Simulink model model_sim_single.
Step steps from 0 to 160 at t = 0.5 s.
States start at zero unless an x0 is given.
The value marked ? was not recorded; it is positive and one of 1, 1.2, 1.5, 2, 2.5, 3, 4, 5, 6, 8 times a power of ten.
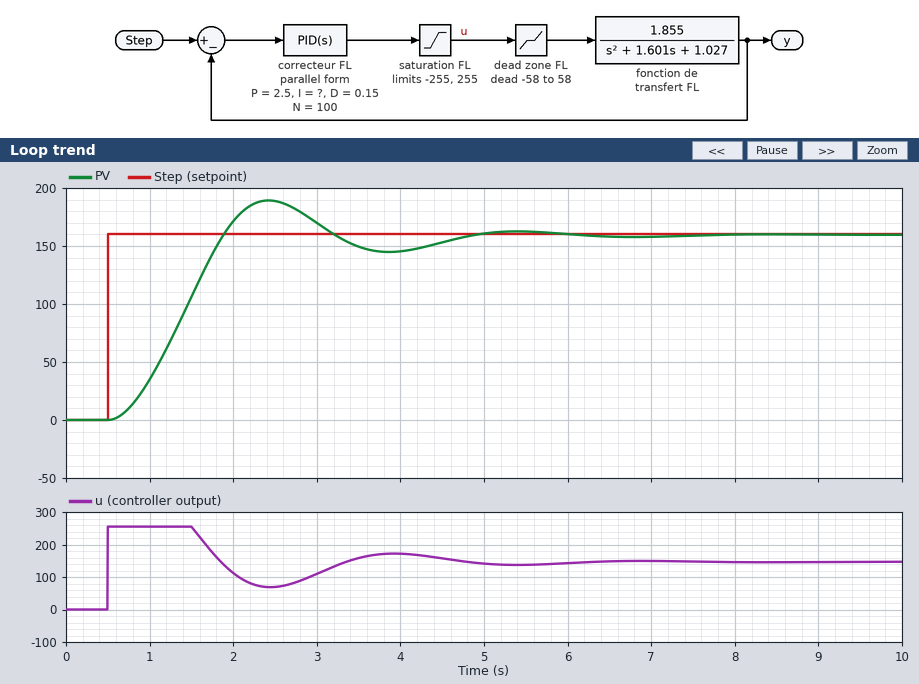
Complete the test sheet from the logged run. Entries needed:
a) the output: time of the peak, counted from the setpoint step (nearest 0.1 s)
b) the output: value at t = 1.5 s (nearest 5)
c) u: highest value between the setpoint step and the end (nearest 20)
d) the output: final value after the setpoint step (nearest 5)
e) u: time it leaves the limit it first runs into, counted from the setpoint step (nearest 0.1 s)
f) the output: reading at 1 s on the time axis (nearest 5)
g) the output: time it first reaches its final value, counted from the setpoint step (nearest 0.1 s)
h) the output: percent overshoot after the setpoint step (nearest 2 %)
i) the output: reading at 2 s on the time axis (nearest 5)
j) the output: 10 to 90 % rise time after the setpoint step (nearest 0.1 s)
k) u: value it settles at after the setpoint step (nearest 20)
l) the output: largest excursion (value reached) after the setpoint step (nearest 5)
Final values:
1.9 s
105
260
160
1.0 s
35
1.4 s
18 %
170
0.9 s
140
190
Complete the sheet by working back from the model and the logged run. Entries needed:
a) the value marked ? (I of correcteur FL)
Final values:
1.2
